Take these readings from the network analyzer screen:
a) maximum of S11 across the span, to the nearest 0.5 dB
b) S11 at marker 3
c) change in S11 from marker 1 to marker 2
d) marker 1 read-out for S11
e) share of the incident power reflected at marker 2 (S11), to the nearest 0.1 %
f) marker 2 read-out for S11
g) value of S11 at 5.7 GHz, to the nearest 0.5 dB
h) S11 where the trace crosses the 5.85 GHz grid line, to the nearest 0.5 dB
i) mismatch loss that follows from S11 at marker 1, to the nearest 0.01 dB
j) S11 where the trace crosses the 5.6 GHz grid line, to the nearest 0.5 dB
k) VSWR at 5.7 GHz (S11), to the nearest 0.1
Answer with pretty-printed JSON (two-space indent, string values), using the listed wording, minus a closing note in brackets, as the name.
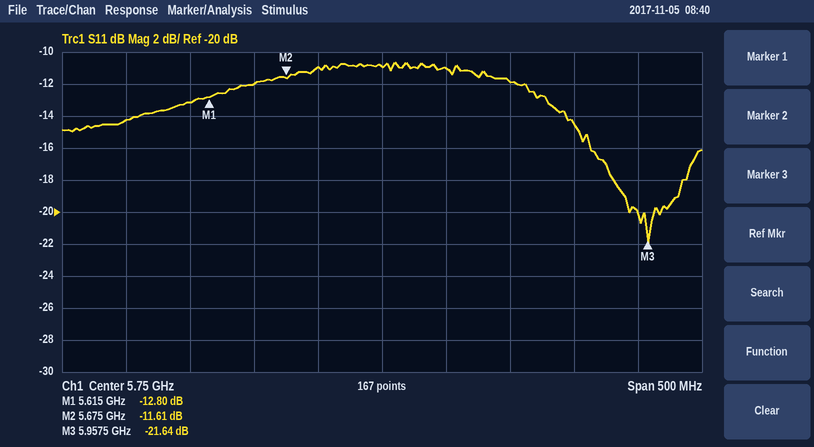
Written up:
{
  "maximum of S11 across the span, to the nearest 0.5 dB": "-10.5 dB",
  "S11 at marker 3": "-21.64 dB",
  "change in S11 from marker 1 to marker 2": "1.19 dB",
  "marker 1 read-out for S11": "-12.80 dB",
  "share of the incident power reflected at marker 2 (S11), to the nearest 0.1 %": "6.9 %",
  "marker 2 read-out for S11": "-11.61 dB",
  "value of S11 at 5.7 GHz, to the nearest 0.5 dB": "-11.0 dB",
  "S11 where the trace crosses the 5.85 GHz grid line, to the nearest 0.5 dB": "-12.0 dB",
  "mismatch loss that follows from S11 at marker 1, to the nearest 0.01 dB": "0.23 dB",
  "S11 where the trace crosses the 5.6 GHz grid line, to the nearest 0.5 dB": "-13.0 dB",
  "VSWR at 5.7 GHz (S11), to the nearest 0.1": "1.8"
}
